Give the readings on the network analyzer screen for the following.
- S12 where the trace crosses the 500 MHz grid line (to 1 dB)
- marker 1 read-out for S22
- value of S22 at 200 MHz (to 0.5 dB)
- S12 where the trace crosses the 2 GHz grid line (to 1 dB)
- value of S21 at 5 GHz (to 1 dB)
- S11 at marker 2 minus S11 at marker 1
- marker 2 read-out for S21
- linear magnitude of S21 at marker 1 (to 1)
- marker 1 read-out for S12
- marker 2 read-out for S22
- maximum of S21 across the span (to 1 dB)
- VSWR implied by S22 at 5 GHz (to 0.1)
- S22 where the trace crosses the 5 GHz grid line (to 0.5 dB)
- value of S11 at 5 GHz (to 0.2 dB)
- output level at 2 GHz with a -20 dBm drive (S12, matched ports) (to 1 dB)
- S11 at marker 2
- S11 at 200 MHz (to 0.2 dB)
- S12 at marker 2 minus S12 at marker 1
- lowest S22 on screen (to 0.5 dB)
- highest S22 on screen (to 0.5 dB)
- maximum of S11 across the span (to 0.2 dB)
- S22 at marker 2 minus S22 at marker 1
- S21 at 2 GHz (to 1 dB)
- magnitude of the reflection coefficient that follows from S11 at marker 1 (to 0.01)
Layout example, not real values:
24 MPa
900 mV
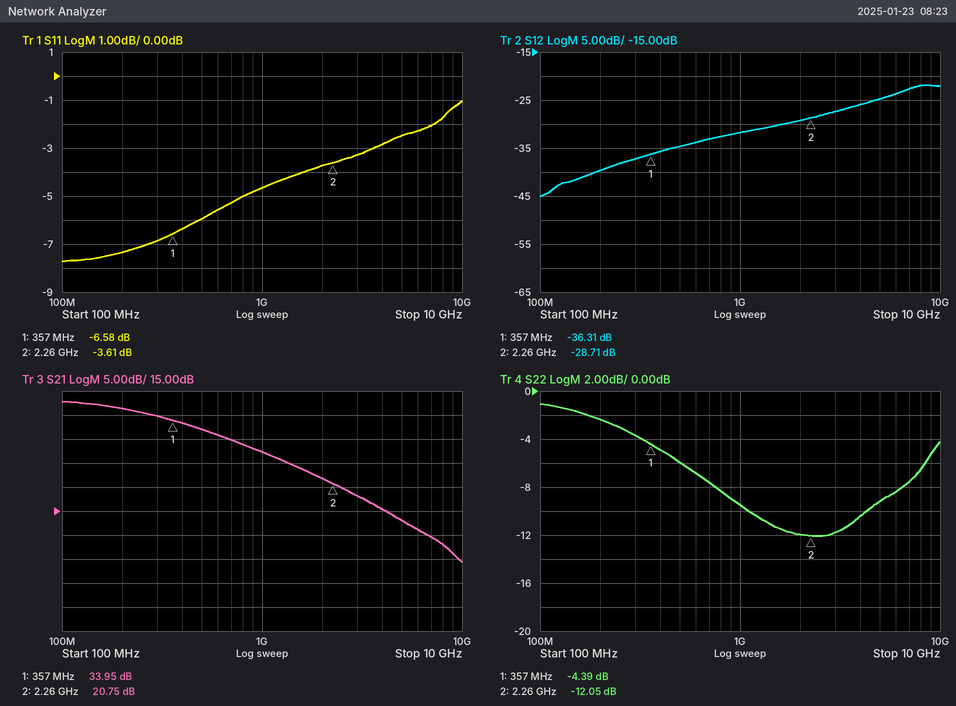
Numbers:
-35 dB
-4.39 dB
-2.5 dB
-29 dB
13 dB
2.97 dB
20.75 dB
50
-36.31 dB
-12.05 dB
38 dB
2.1
-9.0 dB
-2.4 dB
-49 dBm
-3.61 dB
-7.4 dB
7.60 dB
-12.0 dB
-1.0 dB
-1.0 dB
-7.66 dB
22 dB
0.47
